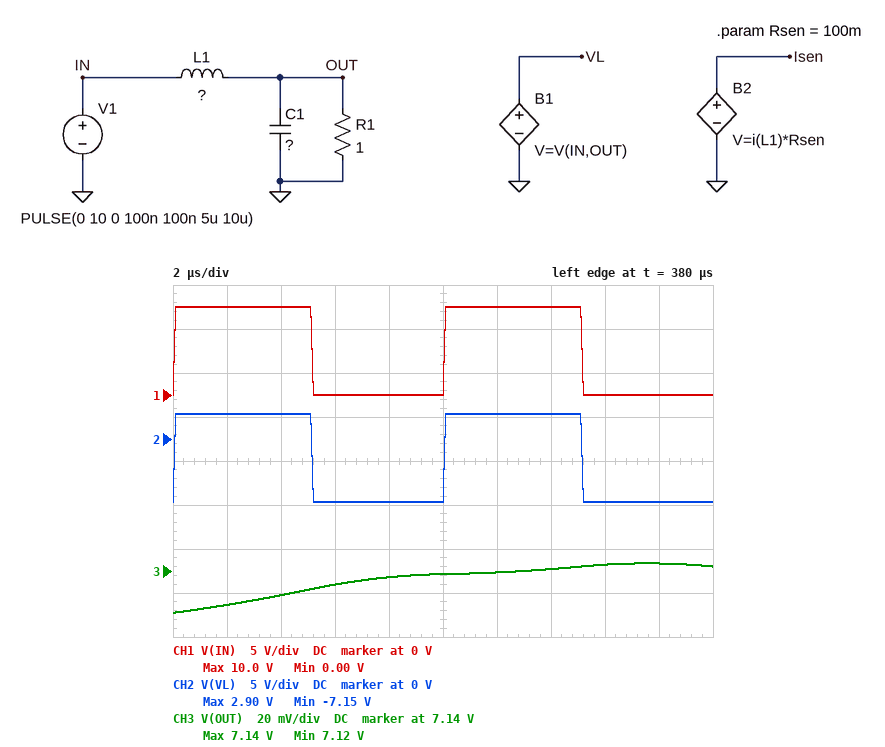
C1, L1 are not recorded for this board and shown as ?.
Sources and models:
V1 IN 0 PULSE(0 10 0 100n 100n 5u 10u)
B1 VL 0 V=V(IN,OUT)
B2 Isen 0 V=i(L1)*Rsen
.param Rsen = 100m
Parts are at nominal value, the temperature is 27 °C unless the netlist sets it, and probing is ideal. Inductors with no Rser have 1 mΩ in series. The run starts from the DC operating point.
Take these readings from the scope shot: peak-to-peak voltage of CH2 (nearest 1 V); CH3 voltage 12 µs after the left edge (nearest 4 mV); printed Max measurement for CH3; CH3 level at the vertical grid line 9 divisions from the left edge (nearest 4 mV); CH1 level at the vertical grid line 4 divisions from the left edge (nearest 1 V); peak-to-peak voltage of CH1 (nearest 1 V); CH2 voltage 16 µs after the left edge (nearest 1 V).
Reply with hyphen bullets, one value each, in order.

- 10 V
- 7.140 V
- 7.14 V
- 7.144 V
- 0 V
- 10 V
- -7 V
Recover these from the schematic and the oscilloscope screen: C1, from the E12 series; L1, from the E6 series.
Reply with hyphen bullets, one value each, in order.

- 220 µF
- 68 µH
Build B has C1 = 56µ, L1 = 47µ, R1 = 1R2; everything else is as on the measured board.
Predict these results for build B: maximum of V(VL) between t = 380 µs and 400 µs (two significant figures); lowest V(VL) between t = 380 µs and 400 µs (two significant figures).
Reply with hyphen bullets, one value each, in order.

- 5.2 V
- -4.9 V
